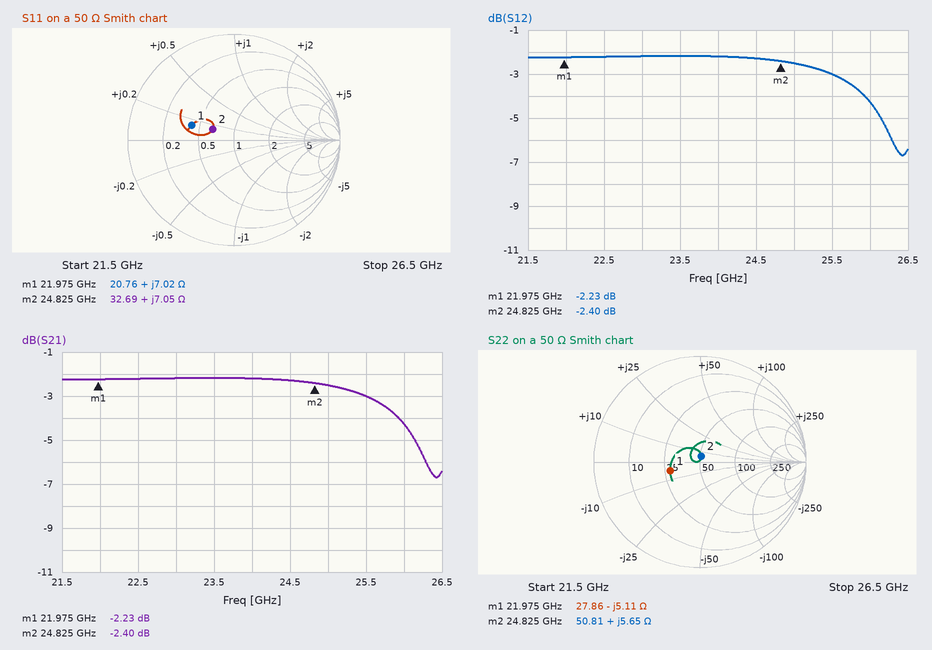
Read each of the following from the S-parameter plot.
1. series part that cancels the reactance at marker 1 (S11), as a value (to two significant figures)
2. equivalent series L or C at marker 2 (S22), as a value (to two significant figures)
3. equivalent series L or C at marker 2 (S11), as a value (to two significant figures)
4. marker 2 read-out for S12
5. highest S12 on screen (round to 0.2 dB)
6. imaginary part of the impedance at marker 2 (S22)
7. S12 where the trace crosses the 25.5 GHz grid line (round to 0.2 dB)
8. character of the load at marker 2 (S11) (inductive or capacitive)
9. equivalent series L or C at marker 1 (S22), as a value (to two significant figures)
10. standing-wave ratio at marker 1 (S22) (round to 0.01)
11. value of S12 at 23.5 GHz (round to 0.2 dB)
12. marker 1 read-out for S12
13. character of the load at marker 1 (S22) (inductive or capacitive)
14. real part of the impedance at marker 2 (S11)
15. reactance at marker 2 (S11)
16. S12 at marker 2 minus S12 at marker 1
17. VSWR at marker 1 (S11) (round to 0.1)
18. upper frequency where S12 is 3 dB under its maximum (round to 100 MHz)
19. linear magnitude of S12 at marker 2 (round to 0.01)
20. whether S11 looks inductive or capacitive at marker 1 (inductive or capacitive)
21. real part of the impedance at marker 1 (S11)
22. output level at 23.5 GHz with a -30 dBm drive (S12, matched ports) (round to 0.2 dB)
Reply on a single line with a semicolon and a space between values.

1.0 pF; 36 pH; 45 pH; -2.40 dB; -2.2 dB; +5.65 Ω; -3.0 dB; inductive; 1.4 pF; 1.82; -2.2 dB; -2.23 dB; capacitive; 32.69 Ω; +7.05 Ω; -0.17 dB; 2.5; 26.2 GHz; 0.76; inductive; 20.76 Ω; -32.2 dBm
